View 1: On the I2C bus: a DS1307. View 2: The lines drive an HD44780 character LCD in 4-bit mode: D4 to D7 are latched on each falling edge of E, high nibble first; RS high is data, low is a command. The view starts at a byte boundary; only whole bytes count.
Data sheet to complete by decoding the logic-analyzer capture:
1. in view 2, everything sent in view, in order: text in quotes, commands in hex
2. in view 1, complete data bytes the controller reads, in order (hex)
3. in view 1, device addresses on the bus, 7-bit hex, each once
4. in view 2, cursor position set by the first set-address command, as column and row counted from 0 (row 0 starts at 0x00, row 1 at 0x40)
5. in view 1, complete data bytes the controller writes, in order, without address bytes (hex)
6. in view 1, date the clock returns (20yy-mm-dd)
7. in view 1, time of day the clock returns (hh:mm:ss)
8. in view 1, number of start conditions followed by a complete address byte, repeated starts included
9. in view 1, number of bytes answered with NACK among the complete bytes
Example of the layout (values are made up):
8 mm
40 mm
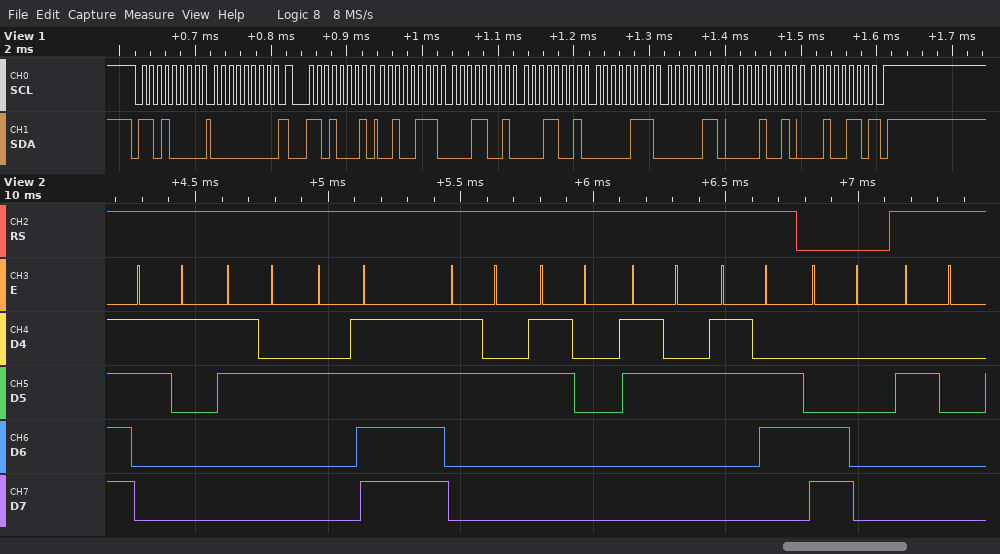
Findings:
"12/2026" 0xC0 " "
27 19 19 07 06 12 26
0x68
column 0, row 1
00
2026-12-06
19:19:27
2
1
